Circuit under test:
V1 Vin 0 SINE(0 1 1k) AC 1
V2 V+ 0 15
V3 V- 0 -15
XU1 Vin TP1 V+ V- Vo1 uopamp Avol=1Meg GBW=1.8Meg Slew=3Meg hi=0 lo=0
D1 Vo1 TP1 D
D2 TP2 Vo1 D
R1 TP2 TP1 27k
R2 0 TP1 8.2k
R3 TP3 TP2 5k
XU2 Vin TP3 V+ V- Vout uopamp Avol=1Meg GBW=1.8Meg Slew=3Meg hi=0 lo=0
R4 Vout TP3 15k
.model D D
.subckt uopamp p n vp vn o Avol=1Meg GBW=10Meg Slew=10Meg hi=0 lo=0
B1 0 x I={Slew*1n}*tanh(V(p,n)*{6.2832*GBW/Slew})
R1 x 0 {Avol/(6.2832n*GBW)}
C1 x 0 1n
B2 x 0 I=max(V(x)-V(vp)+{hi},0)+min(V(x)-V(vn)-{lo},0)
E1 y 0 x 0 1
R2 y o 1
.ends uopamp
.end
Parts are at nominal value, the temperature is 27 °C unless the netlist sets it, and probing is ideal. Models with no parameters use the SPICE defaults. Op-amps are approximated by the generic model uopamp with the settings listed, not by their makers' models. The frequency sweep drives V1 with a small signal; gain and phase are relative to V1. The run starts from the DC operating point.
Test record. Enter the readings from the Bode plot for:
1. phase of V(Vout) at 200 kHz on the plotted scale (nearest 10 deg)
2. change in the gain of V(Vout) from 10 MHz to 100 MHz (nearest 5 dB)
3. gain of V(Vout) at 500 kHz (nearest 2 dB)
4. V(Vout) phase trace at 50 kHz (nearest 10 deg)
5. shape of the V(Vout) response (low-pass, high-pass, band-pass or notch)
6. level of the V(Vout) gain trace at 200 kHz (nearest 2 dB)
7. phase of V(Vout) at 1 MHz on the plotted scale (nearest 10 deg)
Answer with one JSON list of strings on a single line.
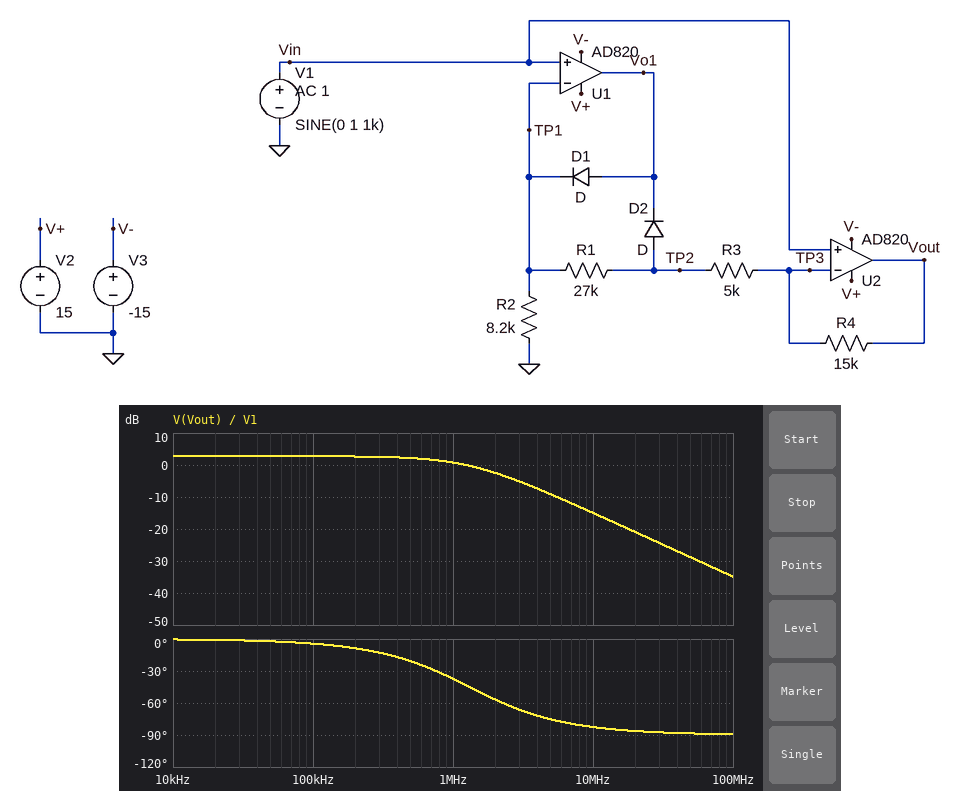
["-10 deg", "-20 dB", "2 dB", "0 deg", "low-pass", "2 dB", "-40 deg"]
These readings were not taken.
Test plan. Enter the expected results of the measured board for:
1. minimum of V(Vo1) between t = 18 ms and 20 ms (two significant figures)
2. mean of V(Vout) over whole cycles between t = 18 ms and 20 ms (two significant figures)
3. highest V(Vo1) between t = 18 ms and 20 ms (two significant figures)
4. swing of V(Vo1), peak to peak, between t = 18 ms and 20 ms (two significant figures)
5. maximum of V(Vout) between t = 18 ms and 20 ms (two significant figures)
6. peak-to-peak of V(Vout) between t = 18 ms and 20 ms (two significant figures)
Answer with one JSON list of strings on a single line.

["-4.9 V", "3.1 V", "1.6 V", "6.5 V", "8.9 V", "8.9 V"]
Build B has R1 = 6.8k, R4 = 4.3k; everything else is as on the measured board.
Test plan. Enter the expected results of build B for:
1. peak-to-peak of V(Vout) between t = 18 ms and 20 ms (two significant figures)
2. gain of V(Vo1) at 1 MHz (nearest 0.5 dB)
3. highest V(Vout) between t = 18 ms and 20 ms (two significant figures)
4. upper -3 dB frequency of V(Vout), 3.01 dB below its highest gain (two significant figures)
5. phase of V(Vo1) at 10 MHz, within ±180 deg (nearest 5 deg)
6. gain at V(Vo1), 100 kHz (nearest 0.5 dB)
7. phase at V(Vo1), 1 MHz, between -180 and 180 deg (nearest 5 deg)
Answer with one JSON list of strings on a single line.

["1.3 V", "2.5 dB", "1.0 V", "1.5 MHz", "-85 deg", "20.5 dB", "-75 deg"]
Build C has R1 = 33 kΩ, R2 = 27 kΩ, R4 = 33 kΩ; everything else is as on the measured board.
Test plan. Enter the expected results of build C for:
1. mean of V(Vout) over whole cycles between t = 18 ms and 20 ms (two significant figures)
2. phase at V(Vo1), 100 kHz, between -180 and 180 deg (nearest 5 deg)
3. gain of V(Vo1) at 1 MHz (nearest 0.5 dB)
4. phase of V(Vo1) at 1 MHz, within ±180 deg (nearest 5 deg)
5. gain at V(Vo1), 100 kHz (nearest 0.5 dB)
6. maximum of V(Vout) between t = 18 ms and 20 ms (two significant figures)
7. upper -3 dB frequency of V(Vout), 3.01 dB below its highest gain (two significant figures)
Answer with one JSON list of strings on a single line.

["2.6 V", "-85 deg", "3.0 dB", "-75 deg", "20.5 dB", "7.1 V", "1.2 MHz"]
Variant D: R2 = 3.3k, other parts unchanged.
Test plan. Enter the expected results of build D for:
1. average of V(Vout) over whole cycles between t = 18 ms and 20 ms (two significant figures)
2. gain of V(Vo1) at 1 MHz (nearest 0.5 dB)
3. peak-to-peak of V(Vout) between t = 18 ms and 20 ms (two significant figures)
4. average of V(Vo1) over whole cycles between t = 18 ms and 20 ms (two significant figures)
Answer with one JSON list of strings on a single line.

["6.2 V", "4.5 dB", "15 V", "-2.6 V"]
